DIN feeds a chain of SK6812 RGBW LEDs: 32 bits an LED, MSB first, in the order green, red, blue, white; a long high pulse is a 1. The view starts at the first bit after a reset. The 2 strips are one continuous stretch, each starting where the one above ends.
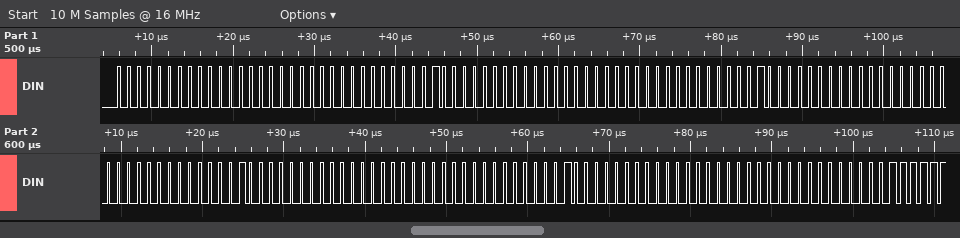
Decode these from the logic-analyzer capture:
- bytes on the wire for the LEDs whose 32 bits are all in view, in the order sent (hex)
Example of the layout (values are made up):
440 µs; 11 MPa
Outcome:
00 00 00 01 00 00 00 01 00 00 00 01 00 00 00 01 00 00 00 01
